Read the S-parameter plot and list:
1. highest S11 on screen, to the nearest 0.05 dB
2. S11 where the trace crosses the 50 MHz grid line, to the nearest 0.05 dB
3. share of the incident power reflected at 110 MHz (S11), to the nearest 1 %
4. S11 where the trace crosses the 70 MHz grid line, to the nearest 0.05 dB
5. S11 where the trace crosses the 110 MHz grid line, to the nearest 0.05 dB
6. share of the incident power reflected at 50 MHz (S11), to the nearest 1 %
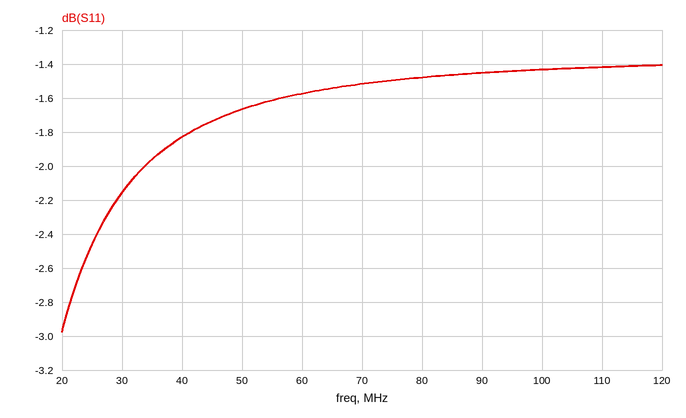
-1.40 dB
-1.65 dB
72 %
-1.50 dB
-1.40 dB
68 %
